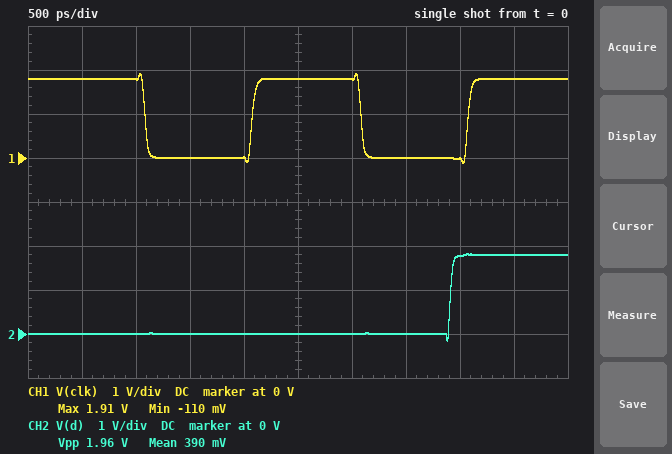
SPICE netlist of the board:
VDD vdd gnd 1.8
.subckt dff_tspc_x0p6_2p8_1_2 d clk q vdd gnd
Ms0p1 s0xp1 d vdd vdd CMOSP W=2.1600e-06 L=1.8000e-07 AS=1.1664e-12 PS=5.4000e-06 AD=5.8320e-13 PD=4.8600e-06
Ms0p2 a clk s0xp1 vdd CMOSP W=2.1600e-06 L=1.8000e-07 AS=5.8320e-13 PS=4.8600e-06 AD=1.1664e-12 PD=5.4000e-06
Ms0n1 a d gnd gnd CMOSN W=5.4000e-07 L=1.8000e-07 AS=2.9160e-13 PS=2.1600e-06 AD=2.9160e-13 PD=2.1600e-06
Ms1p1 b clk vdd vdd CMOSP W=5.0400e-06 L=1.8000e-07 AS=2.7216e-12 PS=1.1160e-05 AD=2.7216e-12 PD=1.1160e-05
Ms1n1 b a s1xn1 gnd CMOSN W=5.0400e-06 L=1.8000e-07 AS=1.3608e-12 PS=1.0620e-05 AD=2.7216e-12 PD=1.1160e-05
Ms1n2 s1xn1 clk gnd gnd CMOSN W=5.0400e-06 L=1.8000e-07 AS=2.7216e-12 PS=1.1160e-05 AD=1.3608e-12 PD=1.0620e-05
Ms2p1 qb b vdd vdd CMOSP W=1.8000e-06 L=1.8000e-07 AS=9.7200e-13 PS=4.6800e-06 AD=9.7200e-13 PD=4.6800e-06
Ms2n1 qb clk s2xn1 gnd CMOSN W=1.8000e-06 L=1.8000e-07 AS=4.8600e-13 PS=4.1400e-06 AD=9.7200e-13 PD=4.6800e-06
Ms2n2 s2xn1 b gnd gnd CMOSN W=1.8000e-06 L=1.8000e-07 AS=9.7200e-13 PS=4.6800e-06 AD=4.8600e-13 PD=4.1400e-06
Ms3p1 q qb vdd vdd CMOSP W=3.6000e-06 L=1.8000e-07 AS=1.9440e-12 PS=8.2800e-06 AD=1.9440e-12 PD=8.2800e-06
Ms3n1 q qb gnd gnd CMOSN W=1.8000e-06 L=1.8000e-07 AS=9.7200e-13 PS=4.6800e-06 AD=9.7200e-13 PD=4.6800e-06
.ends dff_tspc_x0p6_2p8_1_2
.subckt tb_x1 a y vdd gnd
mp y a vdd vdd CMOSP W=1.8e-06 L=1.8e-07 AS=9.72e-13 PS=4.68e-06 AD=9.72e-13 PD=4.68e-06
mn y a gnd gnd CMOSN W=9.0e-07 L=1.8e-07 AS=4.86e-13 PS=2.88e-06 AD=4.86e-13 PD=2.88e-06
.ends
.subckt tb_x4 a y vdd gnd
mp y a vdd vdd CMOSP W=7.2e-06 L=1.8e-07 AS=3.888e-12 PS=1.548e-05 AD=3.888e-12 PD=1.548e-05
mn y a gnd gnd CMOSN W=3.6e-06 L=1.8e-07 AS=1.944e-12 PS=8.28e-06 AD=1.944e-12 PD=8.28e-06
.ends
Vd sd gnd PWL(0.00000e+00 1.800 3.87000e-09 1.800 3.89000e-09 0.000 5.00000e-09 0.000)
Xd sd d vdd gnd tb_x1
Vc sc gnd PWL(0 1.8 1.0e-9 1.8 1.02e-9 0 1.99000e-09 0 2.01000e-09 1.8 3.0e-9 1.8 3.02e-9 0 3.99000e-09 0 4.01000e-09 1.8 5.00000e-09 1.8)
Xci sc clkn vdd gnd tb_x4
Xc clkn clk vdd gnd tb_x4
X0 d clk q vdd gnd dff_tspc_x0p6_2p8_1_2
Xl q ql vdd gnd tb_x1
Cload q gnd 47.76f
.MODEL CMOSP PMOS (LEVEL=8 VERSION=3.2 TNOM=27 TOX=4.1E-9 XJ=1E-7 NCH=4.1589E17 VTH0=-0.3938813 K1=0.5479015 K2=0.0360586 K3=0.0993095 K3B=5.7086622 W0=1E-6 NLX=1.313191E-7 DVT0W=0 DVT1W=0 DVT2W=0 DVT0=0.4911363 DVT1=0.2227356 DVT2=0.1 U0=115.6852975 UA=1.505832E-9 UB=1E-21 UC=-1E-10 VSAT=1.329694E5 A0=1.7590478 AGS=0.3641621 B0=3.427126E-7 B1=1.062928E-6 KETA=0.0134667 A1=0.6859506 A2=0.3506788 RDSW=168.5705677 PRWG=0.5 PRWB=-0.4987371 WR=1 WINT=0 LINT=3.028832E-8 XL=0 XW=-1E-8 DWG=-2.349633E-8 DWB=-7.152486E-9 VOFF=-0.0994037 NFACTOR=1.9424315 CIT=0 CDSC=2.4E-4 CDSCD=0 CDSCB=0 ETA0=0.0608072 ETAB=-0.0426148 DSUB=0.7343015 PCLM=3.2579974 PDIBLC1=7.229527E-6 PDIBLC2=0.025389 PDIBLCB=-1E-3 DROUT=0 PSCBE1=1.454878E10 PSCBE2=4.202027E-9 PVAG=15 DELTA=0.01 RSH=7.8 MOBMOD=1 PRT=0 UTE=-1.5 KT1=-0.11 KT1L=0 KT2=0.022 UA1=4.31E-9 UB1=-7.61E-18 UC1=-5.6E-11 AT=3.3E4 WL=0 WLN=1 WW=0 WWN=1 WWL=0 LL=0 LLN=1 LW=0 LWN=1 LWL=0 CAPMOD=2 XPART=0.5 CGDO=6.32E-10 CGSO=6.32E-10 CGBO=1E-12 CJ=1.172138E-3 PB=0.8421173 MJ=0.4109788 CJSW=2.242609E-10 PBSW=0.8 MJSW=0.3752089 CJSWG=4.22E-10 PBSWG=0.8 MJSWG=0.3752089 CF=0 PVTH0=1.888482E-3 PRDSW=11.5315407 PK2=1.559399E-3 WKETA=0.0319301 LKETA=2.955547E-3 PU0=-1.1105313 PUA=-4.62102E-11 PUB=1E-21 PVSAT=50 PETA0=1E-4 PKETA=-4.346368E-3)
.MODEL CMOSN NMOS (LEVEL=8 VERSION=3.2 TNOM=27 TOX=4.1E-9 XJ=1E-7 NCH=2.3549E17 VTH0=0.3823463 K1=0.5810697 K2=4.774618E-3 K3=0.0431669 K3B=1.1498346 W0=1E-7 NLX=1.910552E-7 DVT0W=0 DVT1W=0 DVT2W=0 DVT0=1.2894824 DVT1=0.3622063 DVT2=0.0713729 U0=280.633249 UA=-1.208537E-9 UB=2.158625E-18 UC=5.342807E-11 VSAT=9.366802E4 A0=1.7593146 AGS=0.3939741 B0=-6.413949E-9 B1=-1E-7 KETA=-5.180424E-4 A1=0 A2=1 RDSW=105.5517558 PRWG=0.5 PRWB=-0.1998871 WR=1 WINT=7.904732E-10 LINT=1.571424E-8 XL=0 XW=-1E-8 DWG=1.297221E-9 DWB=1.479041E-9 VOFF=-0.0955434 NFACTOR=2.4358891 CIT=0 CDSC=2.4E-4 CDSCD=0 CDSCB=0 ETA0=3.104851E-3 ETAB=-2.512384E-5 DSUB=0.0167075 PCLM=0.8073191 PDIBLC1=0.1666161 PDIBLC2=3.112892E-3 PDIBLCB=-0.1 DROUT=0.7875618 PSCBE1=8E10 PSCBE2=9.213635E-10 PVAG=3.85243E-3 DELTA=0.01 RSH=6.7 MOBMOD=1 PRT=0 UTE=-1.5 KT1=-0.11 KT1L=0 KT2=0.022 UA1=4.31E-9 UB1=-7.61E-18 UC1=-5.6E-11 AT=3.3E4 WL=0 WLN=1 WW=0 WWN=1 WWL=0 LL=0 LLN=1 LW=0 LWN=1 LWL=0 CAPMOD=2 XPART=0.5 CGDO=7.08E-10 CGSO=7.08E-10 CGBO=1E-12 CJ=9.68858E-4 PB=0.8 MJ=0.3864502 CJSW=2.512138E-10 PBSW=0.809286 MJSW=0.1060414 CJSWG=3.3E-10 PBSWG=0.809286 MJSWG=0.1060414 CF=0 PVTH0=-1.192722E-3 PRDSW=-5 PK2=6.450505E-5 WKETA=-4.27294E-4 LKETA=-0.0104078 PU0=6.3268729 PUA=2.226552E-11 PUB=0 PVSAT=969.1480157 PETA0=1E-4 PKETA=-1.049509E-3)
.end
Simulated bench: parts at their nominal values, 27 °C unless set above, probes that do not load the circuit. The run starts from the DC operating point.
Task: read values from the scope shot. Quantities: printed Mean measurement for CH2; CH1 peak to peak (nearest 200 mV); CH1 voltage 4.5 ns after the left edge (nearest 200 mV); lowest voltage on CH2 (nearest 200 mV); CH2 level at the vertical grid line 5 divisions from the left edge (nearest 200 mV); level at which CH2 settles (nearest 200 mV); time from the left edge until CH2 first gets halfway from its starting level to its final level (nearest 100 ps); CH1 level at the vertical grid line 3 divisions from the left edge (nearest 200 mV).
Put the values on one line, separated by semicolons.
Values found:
390 mV; 2.0 V; 1.8 V; -200 mV; 0 V; 1.8 V; 3.9 ns; 0 V
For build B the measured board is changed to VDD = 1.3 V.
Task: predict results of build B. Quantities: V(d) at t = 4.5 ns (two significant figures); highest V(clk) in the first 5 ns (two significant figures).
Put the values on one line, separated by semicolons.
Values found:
1.3 V; 1.4 V
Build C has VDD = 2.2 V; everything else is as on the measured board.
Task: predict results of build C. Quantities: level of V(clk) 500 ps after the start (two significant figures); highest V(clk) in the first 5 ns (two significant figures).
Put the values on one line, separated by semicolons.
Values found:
2.2 V; 2.3 V
